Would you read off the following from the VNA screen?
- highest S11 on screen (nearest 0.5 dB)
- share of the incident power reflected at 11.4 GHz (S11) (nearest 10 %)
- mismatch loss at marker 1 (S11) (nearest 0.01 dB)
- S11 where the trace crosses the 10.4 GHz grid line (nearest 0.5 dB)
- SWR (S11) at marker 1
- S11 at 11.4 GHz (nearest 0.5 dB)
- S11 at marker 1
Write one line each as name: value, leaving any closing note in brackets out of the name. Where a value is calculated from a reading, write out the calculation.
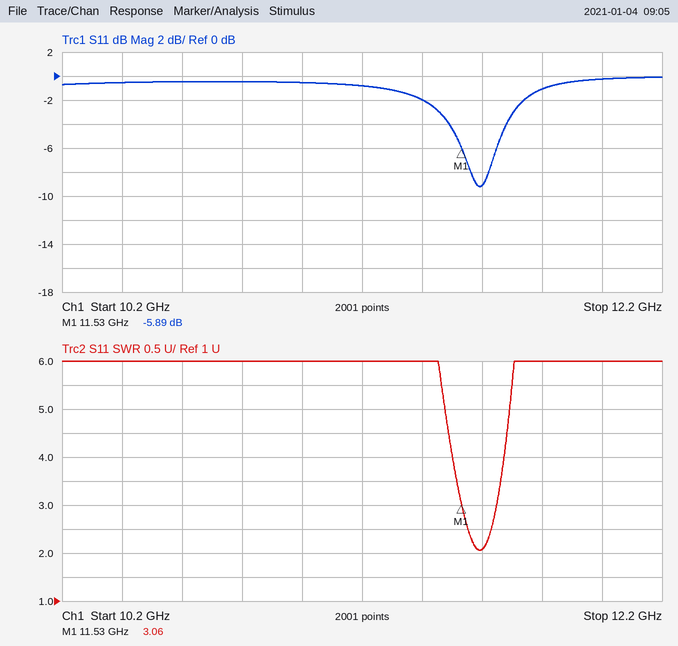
highest S11 on screen: 0.0 dB
share of the incident power reflected at 11.4 GHz (S11): 10^(-2/10) ≈ 63.1 %, so 60 % to the nearest 10 %
mismatch loss at marker 1 (S11): −10 log10(1 − 10^(-5.89/10)) ≈ 1.29 dB
S11 where the trace crosses the 10.4 GHz grid line: -0.5 dB
SWR (S11) at marker 1: 3.06
S11 at 11.4 GHz: -2.0 dB
S11 at marker 1: -5.89 dB
